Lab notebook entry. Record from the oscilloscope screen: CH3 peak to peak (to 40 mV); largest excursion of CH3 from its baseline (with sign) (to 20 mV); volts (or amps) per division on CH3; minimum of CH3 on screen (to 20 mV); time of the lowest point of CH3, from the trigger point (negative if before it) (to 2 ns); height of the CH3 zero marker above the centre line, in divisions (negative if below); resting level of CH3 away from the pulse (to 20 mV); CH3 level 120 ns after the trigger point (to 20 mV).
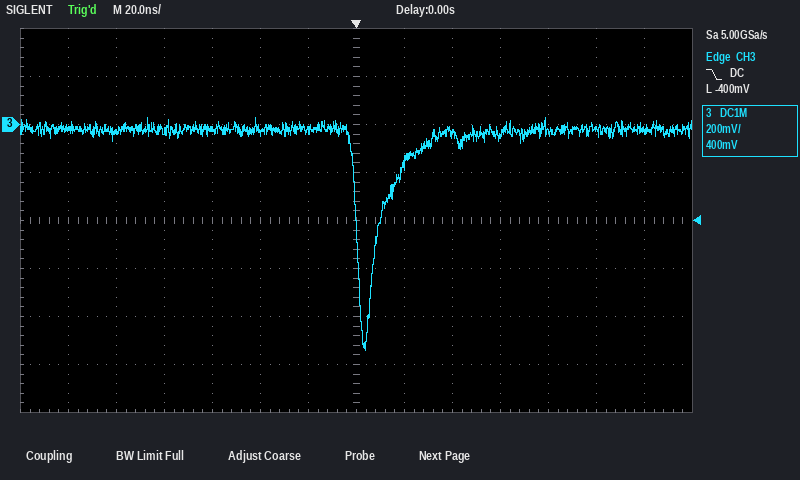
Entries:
960 mV
-920 mV
200 mV
-940 mV
+4 ns
+2.0 div
-20 mV
-20 mV
